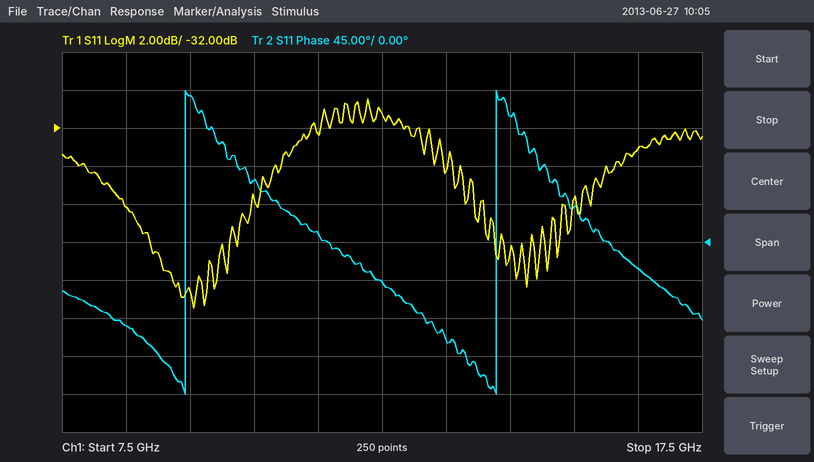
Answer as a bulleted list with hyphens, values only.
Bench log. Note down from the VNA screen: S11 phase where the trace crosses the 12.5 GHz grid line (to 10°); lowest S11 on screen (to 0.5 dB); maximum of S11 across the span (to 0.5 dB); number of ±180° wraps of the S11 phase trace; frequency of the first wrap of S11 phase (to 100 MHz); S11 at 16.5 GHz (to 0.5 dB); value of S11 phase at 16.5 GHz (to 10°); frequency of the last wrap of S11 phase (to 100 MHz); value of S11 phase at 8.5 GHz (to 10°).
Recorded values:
- -50°
- -41.5 dB
- -30.5 dB
- 2
- 9.4 GHz
- -33.0 dB
- -30°
- 14.3 GHz
- -100°
